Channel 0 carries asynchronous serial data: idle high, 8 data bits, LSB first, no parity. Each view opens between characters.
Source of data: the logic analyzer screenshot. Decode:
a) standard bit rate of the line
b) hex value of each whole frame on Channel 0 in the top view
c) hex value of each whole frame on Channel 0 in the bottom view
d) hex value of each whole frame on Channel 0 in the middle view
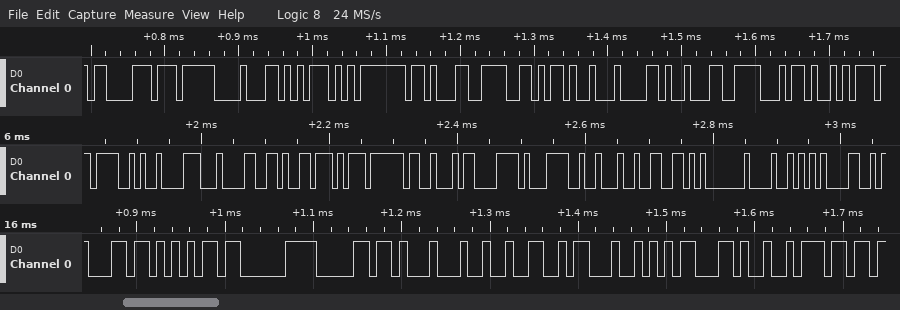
115200 baud
C3, F7, 88, 75, FD, 8B, 9E, 2D, 84, 89, 1E, 4B
6C, B5, E0, B0, 11, 92, 1A, AA, 2C, BA
4F, C2, 84, 96, D7, BF, A2, 78, 3C, 22, 66, 01, 48, 85
